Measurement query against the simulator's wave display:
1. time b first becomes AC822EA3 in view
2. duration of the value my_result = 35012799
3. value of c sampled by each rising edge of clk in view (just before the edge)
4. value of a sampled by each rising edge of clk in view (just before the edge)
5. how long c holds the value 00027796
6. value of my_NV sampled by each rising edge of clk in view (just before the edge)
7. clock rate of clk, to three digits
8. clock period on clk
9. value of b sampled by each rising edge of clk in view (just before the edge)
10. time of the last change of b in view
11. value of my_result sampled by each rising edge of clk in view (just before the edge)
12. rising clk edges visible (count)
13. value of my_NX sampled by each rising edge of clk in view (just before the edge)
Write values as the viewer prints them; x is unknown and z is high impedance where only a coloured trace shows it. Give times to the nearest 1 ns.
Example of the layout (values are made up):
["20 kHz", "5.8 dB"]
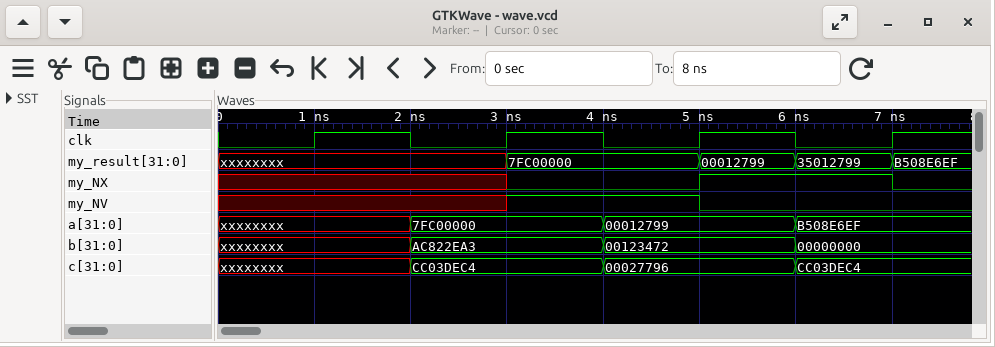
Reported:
["2 ns", "1 ns", "xxxxxxxx, CC03DEC4, 00027796, CC03DEC4", "xxxxxxxx, 7FC00000, 00012799, B508E6EF", "2 ns", "x x 1 0", "500 MHz", "2 ns", "xxxxxxxx, AC822EA3, 00123472, 00000000", "6 ns", "xxxxxxxx, xxxxxxxx, 7FC00000, 35012799", "4", "x x 0 1"]
